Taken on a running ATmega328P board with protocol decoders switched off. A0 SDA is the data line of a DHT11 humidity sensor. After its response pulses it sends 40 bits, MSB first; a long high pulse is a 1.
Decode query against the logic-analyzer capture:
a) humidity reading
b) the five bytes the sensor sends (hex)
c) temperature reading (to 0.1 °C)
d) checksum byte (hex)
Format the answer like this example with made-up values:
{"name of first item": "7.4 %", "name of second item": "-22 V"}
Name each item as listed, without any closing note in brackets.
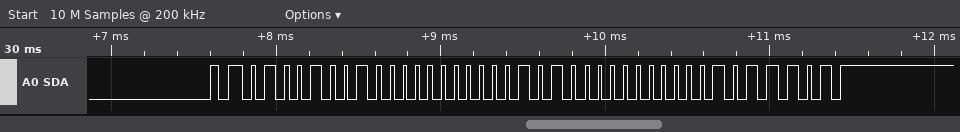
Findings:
{"humidity reading": "73 %", "the five bytes the sensor sends": "49 00 14 00 5D", "temperature reading": "20.0 °C", "checksum byte": "0x5D"}
